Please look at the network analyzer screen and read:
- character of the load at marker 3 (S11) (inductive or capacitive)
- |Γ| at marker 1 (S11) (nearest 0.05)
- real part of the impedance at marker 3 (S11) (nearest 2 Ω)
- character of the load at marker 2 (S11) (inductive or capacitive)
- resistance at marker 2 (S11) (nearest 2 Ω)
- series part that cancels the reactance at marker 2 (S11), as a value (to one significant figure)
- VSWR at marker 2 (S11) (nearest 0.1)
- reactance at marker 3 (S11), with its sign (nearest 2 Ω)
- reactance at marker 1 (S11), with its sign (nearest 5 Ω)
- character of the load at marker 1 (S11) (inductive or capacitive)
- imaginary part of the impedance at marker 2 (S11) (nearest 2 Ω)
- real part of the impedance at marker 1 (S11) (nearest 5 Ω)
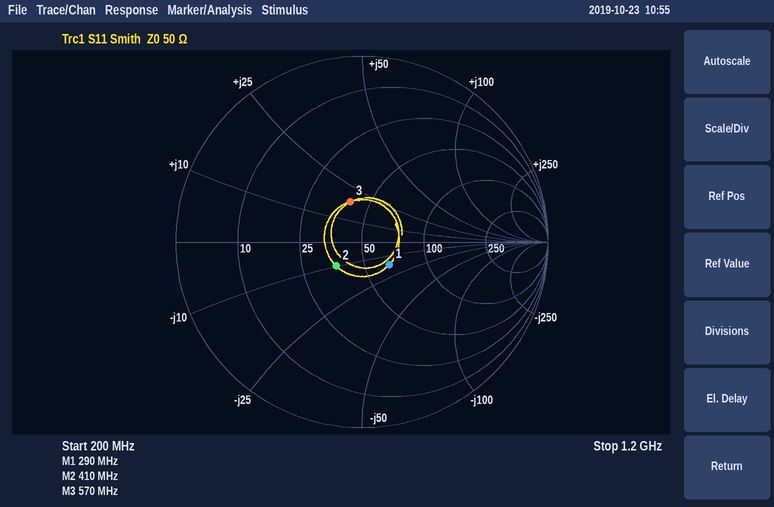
inductive
0.20
40 Ω
capacitive
36 Ω
4 nH
1.5
+18 Ω
-15 Ω
capacitive
-10 Ω
65 Ω
